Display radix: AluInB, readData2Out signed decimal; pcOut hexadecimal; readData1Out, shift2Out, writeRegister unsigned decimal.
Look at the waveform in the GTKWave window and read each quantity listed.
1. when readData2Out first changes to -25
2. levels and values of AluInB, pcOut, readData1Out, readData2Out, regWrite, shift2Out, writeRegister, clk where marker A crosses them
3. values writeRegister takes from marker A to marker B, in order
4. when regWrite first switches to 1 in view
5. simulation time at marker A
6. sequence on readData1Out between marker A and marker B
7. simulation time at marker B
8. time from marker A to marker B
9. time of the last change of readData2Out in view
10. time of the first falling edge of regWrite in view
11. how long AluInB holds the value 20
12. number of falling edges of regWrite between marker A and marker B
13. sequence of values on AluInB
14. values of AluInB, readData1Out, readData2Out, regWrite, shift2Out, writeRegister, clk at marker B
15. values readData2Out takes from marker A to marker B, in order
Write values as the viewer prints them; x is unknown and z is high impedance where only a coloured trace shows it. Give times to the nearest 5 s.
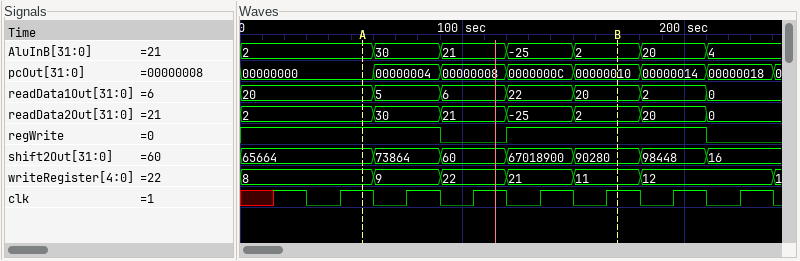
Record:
120 s
AluInB=2, pcOut=00000000, readData1Out=20, readData2Out=2, regWrite=1, shift2Out=65664, writeRegister=8, clk=1
8, 9, 22, 21, 11
120 s
55 s
20, 5, 6, 22, 20
170 s
115 s
210 s
90 s
30 s
1
2, 30, 21, -25, 2, 20, 4
AluInB=2, readData1Out=20, readData2Out=2, regWrite=1, shift2Out=90280, writeRegister=11, clk=1
2, 30, 21, -25, 2
